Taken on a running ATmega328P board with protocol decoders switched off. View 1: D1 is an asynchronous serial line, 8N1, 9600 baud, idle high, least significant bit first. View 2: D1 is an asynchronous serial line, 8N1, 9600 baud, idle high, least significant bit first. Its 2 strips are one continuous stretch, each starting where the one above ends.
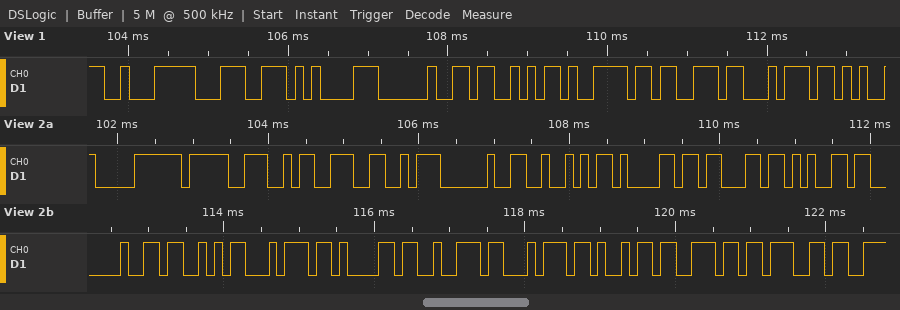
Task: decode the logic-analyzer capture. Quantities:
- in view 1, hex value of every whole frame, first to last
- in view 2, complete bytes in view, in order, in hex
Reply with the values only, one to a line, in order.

E2 9C 85 20 53 79 73 74
F0 9F 9A A6 20 52 61 63 65 20 53 74 61 72 74 69 6E 67
